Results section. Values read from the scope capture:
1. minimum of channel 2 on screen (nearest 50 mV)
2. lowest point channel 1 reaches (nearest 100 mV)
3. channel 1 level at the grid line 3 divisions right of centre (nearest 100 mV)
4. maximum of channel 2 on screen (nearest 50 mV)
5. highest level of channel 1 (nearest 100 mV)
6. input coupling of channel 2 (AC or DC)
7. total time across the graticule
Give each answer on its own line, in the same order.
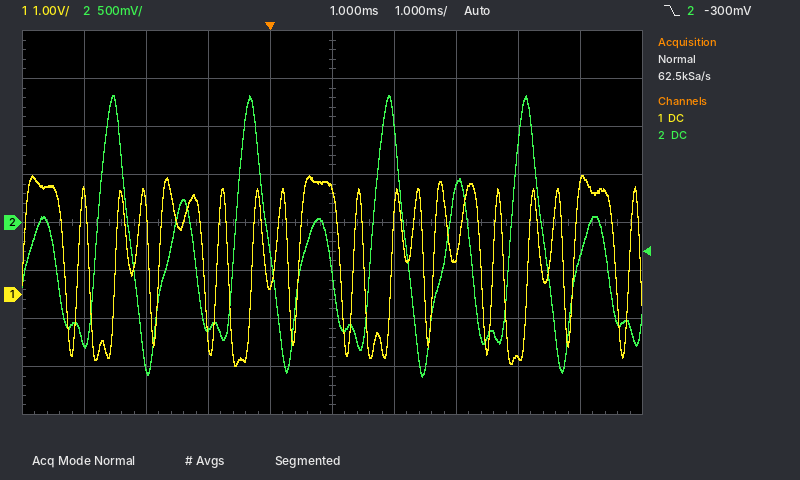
-1.60 V
-1.5 V
-1.3 V
1.30 V
2.5 V
DC
10 ms
